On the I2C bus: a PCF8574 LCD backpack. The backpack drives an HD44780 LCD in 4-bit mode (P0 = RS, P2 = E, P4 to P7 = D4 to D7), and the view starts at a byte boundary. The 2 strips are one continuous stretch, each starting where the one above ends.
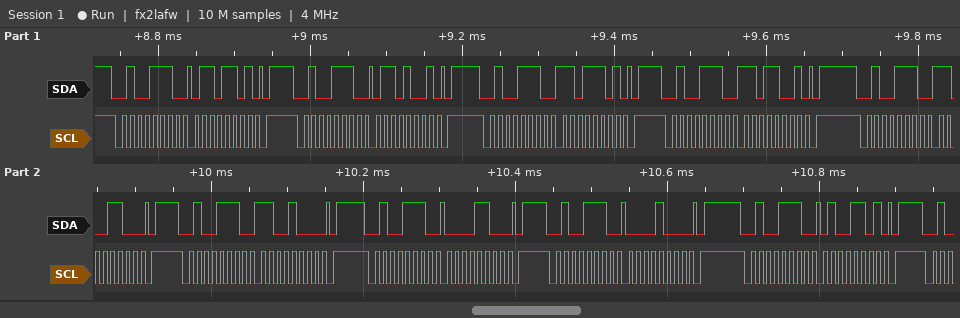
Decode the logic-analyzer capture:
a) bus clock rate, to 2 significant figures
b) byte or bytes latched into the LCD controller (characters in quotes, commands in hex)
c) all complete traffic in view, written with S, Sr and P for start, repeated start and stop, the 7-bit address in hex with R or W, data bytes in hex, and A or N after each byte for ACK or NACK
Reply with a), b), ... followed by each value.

a) 100 kHz
b) 'm' 0xC0
c) S 27W A 6D A P S 27W A 69 A P S 27W A DD A P S 27W A D9 A P S 27W A CC A P S 27W A C8 A P S 27W A 0C A P S 27W A 08 A P S 27W A 4D A P
